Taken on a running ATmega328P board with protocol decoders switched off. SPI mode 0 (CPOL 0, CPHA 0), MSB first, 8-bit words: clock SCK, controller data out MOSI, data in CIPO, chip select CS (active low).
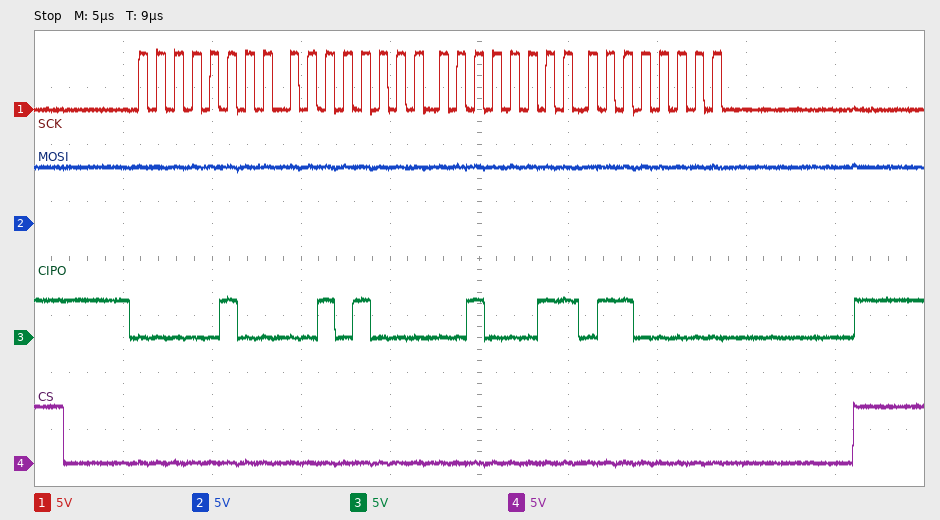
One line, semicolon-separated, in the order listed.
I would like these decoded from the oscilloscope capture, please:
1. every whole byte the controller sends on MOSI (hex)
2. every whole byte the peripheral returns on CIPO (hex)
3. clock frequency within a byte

FF FF FF FF; 04 28 23 60; 1 MHz
